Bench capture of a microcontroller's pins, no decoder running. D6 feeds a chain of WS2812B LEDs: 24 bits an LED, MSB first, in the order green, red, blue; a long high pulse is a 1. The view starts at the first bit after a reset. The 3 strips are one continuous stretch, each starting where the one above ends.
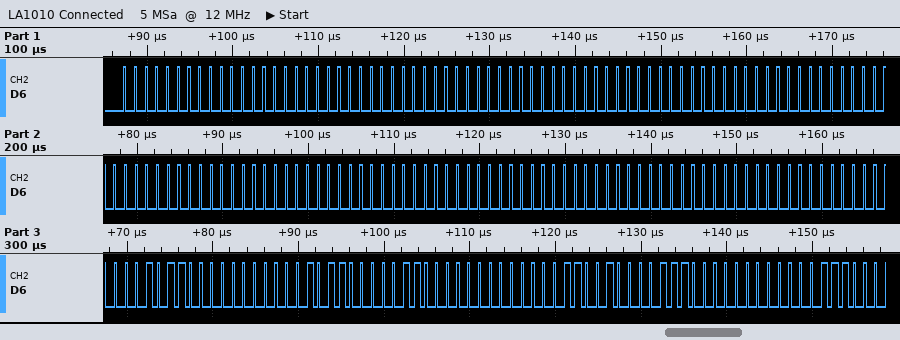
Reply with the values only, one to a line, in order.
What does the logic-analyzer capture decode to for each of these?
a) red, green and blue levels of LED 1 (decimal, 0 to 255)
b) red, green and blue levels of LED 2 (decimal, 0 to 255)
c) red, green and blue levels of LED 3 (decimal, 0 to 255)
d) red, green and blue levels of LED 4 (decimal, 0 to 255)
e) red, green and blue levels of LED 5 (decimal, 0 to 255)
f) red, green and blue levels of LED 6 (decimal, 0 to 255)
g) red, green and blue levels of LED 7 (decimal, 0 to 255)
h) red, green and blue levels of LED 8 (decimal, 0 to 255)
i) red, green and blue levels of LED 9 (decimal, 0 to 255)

0, 0, 0
0, 0, 0
0, 0, 0
0, 0, 0
0, 0, 0
0, 0, 0
0, 11, 22
0, 12, 25
0, 14, 28
